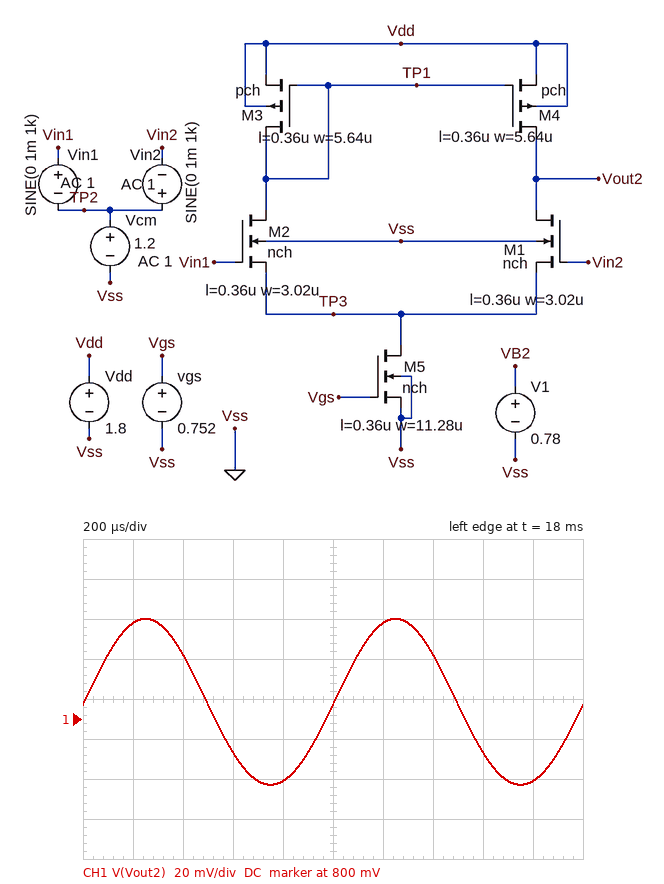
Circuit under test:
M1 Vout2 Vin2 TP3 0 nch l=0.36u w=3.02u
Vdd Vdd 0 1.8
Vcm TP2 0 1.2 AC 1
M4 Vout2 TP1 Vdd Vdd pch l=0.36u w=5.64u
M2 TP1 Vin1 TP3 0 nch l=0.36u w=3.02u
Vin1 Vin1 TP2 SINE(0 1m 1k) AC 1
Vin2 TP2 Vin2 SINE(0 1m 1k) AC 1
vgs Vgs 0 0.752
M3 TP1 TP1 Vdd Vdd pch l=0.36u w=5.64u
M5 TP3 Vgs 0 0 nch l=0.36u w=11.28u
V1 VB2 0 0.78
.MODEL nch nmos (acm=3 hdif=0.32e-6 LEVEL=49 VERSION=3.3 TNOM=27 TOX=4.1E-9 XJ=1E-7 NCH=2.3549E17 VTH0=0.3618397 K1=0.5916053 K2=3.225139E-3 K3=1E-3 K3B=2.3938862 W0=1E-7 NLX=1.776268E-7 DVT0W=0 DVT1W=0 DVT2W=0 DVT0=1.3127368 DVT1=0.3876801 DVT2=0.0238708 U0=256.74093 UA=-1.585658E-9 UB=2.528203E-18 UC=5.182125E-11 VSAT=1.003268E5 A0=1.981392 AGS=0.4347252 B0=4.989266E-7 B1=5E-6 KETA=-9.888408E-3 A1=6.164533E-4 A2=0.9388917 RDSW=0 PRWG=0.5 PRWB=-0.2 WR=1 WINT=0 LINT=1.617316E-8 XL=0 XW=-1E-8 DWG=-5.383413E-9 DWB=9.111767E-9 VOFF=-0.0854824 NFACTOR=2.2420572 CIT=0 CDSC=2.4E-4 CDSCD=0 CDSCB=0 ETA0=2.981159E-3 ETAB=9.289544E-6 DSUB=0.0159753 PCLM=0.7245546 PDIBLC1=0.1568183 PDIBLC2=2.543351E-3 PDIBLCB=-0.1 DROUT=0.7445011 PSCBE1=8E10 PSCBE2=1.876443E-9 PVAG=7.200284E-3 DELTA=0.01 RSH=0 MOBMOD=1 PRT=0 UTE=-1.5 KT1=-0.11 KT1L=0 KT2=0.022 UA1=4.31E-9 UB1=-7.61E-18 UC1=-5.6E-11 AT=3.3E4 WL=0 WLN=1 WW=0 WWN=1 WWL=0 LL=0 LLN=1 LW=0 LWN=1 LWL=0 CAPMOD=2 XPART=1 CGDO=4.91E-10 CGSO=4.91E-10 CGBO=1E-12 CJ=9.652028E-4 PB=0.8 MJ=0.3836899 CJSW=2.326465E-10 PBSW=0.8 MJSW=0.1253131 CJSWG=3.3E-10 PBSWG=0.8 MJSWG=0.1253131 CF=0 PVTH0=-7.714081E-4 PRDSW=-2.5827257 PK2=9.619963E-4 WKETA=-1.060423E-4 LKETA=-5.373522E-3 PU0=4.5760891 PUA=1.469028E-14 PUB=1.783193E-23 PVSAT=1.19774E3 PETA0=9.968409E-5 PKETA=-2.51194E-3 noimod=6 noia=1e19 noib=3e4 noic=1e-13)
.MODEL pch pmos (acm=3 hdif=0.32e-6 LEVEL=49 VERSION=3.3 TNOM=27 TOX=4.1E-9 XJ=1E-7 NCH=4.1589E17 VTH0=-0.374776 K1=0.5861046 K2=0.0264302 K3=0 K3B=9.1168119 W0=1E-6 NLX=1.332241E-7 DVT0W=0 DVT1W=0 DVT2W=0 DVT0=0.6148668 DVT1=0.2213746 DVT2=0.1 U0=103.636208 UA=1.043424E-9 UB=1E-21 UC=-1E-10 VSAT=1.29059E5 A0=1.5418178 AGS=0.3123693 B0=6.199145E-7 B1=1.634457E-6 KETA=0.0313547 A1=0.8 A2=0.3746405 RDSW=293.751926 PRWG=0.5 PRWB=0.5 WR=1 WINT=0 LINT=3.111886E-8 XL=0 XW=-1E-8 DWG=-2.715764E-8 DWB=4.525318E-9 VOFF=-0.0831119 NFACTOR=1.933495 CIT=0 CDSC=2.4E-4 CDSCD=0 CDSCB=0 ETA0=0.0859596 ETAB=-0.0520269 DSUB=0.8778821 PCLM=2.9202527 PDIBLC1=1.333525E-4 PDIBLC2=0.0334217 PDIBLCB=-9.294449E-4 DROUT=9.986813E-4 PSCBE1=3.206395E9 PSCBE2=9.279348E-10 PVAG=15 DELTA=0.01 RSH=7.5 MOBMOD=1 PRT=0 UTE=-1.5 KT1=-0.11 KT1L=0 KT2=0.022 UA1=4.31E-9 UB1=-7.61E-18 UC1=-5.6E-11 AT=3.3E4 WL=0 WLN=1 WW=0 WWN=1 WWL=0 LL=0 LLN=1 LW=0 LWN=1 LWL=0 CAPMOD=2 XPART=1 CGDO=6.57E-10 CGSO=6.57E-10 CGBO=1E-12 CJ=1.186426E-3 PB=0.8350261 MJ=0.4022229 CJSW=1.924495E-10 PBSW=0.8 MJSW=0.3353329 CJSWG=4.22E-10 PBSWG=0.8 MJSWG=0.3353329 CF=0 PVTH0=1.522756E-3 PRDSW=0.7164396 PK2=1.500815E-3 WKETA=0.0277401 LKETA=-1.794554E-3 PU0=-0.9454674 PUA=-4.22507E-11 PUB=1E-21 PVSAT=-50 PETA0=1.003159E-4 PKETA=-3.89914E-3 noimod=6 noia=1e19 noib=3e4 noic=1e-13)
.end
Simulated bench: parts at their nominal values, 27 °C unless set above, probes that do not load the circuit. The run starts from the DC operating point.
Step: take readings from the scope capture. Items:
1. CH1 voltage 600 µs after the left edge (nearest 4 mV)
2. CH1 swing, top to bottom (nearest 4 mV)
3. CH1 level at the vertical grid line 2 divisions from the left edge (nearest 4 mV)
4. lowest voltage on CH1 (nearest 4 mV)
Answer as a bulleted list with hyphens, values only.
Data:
- 784 mV
- 84 mV
- 832 mV
- 768 mV
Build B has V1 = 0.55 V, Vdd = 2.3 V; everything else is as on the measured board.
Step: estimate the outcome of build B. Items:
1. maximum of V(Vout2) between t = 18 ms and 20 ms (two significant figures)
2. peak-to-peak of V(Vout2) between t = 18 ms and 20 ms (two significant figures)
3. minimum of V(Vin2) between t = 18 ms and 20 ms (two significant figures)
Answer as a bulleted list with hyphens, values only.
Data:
- 1.4 V
- 120 mV
- 1.2 V
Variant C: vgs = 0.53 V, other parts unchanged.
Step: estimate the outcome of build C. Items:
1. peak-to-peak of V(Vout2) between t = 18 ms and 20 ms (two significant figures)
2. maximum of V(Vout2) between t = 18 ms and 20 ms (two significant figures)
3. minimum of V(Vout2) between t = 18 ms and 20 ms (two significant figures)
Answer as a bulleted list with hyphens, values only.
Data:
- 160 mV
- 1.3 V
- 1.1 V
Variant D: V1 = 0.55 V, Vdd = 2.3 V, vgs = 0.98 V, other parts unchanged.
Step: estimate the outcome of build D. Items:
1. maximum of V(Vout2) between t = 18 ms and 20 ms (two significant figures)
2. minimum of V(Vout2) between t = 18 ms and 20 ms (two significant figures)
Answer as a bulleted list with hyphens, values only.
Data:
- 1.1 V
- 1.0 V
